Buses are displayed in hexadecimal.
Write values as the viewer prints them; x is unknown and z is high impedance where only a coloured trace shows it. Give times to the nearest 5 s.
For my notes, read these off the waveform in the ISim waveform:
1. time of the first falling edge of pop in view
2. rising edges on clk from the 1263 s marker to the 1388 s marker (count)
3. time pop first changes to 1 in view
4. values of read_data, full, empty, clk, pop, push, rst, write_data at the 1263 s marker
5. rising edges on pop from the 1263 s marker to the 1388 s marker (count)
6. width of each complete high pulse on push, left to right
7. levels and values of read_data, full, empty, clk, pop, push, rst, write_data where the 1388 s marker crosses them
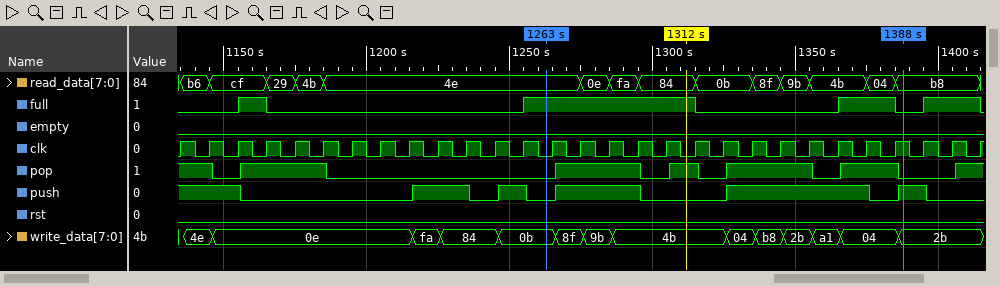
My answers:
1145 s
13
1155 s
read_data=4e, full=1, empty=0, clk=0, pop=0, push=0, rst=0, write_data=0b
4
20 s, 10 s, 30 s, 50 s, 10 s
read_data=b8, full=0, empty=0, clk=1, pop=0, push=1, rst=0, write_data=2b
